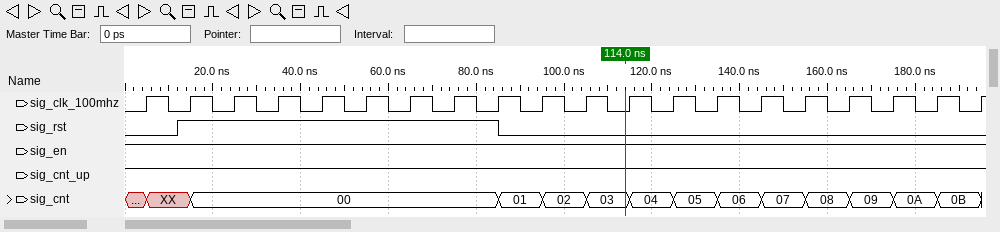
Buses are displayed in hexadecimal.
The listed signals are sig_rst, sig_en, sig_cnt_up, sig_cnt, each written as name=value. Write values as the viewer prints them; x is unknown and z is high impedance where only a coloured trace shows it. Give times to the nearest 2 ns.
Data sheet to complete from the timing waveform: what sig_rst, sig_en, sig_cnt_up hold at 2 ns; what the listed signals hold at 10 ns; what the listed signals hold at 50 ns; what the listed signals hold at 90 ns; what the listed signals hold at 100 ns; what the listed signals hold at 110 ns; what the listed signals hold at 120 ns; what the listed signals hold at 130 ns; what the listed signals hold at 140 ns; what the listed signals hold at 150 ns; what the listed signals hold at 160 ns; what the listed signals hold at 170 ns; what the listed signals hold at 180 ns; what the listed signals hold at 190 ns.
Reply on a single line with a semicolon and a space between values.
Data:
sig_rst=0, sig_en=1, sig_cnt_up=1; sig_rst=0, sig_en=1, sig_cnt_up=1, sig_cnt=XX; sig_rst=1, sig_en=1, sig_cnt_up=1, sig_cnt=00; sig_rst=0, sig_en=1, sig_cnt_up=1, sig_cnt=01; sig_rst=0, sig_en=1, sig_cnt_up=1, sig_cnt=02; sig_rst=0, sig_en=1, sig_cnt_up=1, sig_cnt=03; sig_rst=0, sig_en=1, sig_cnt_up=1, sig_cnt=04; sig_rst=0, sig_en=1, sig_cnt_up=1, sig_cnt=05; sig_rst=0, sig_en=1, sig_cnt_up=1, sig_cnt=06; sig_rst=0, sig_en=1, sig_cnt_up=1, sig_cnt=07; sig_rst=0, sig_en=1, sig_cnt_up=1, sig_cnt=08; sig_rst=0, sig_en=1, sig_cnt_up=1, sig_cnt=09; sig_rst=0, sig_en=1, sig_cnt_up=1, sig_cnt=0A; sig_rst=0, sig_en=1, sig_cnt_up=1, sig_cnt=0B
